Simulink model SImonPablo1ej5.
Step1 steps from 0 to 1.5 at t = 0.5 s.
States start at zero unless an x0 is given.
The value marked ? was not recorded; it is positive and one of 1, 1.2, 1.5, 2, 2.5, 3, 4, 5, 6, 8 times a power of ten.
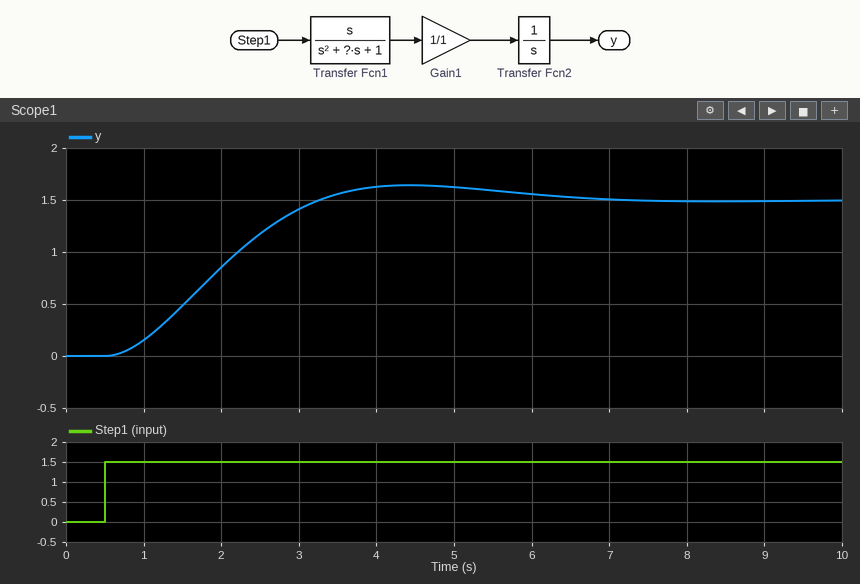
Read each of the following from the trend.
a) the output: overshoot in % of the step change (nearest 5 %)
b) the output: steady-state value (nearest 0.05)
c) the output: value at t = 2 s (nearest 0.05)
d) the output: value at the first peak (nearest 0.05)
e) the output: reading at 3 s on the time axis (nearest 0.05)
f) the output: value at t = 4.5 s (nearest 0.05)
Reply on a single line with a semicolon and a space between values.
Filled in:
10 %; 1.50; 0.85; 1.65; 1.40; 1.65
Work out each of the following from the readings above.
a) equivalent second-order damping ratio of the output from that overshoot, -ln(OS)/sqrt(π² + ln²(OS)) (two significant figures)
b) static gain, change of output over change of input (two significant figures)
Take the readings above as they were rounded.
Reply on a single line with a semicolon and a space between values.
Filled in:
0.59; 1.0
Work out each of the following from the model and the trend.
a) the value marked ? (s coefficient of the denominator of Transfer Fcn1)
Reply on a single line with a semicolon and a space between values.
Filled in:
1.2
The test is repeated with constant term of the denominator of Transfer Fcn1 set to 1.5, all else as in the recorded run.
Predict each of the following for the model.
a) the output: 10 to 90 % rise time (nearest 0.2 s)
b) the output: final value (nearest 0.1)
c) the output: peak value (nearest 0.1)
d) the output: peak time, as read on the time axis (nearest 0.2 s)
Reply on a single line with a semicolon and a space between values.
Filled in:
1.4 s; 1.0; 1.2; 3.4 s
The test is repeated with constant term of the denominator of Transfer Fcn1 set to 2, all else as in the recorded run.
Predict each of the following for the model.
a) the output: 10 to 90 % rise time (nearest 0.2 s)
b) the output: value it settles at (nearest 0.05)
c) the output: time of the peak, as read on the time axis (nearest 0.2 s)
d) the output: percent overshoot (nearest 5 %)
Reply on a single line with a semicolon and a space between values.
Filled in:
1.0 s; 0.75; 3.0 s; 25 %
